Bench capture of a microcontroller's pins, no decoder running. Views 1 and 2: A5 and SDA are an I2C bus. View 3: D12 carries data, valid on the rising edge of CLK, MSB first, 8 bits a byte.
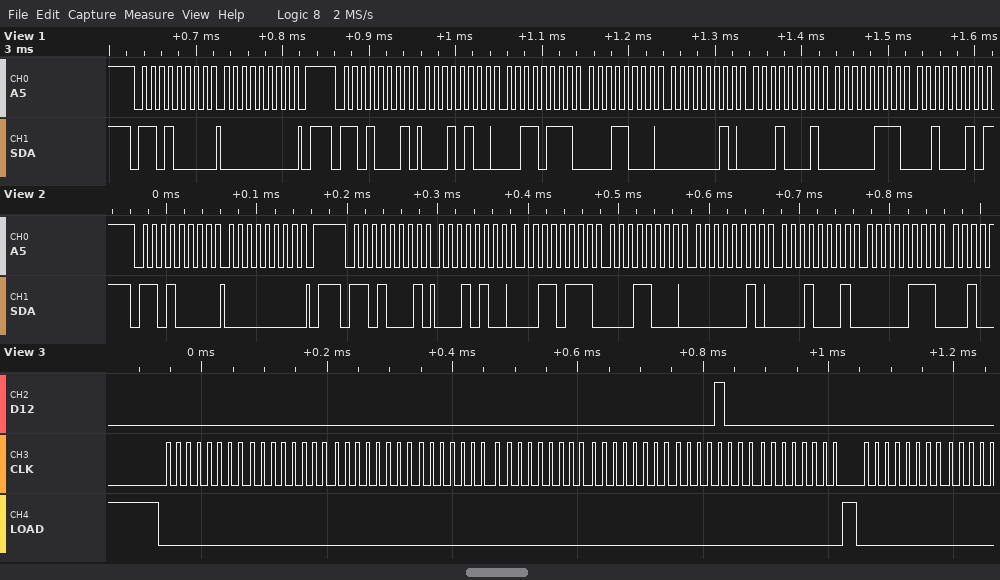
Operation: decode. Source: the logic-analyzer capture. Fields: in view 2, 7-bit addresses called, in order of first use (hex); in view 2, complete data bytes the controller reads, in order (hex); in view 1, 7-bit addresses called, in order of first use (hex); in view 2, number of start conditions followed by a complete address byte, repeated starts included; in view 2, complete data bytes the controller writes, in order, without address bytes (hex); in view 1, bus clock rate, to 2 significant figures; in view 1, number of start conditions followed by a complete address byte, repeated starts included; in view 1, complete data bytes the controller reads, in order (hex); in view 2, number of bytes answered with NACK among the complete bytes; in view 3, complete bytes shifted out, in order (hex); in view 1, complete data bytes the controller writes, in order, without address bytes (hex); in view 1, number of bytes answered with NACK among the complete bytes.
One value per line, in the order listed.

0x68
14 37 18 02 11 07
0x68
2
00
100 kHz
2
14 37 18 02 11 07 22
0
00 00 00 00 00 00 08 00 00
00
1
